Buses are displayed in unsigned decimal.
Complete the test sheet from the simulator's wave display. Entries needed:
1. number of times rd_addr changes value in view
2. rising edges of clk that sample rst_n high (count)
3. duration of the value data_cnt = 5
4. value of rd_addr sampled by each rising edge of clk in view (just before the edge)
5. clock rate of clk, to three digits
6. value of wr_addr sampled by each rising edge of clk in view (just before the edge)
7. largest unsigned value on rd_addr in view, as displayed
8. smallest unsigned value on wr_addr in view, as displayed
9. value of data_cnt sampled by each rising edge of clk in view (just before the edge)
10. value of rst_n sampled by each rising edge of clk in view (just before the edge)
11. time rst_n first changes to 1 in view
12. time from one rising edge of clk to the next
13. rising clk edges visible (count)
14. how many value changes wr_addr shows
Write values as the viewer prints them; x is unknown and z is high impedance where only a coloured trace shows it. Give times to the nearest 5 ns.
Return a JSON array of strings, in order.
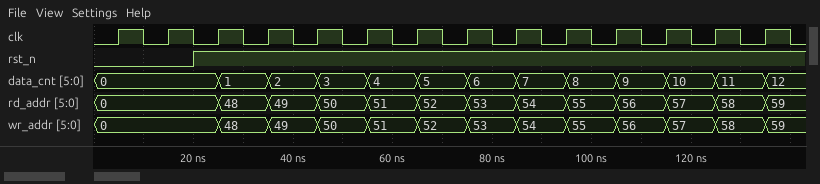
["12", "12", "10 ns", "0, 0, 0, 48, 49, 50, 51, 52, 53, 54, 55, 56, 57, 58", "100 MHz", "0, 0, 0, 48, 49, 50, 51, 52, 53, 54, 55, 56, 57, 58", "59", "0", "0, 0, 0, 1, 2, 3, 4, 5, 6, 7, 8, 9, 10, 11", "0 0 1 1 1 1 1 1 1 1 1 1 1 1", "20 ns", "10 ns", "14", "12"]
